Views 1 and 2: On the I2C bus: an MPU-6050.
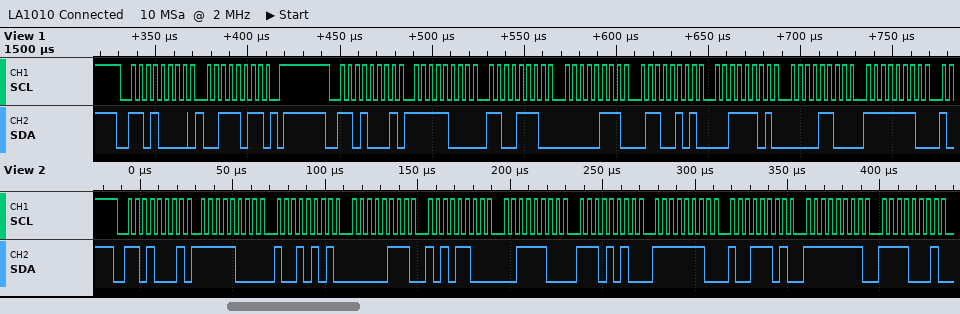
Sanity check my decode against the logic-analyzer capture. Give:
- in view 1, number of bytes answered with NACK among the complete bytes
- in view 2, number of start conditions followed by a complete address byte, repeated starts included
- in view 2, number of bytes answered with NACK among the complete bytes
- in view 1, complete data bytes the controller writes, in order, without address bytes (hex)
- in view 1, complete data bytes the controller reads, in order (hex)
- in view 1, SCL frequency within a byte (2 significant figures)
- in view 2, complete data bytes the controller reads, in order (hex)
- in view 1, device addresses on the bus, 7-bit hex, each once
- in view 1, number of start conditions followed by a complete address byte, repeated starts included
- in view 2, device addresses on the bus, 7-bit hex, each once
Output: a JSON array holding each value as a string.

["0", "1", "0", "3B", "F8 CE 07 65 3D 0C FE", "250 kHz", "F8 95 07 AC 3C EA FE 9D FF F1", "0x68", "2", "0x68"]
